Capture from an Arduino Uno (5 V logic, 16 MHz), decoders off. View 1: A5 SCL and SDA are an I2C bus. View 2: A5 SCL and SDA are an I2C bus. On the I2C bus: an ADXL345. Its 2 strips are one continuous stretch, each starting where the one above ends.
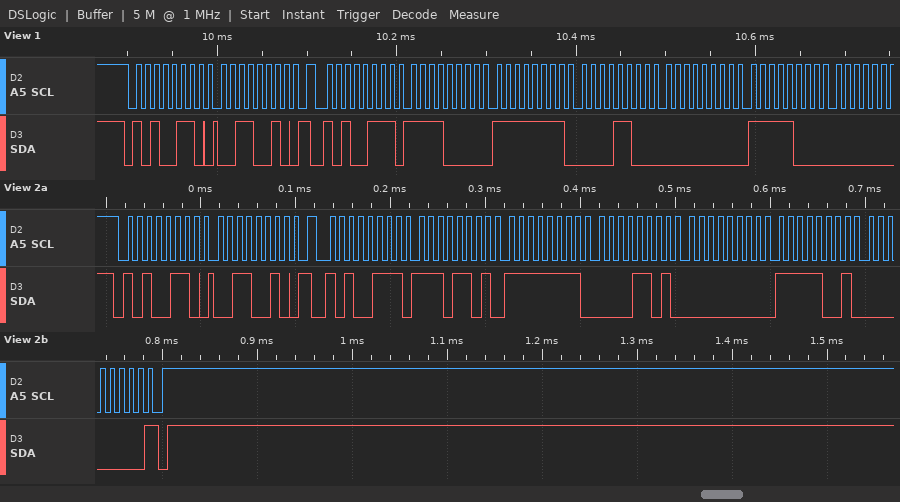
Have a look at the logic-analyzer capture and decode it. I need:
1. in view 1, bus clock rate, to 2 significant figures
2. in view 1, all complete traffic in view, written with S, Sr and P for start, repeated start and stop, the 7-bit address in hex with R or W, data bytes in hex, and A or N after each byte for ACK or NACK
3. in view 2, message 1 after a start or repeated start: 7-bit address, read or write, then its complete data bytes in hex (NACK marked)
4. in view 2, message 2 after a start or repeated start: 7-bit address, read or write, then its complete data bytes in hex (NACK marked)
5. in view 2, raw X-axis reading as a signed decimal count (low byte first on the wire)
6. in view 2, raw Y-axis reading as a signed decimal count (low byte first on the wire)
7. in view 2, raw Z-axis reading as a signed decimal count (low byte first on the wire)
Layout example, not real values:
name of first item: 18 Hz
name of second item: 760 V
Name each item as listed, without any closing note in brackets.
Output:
in view 1, bus clock rate, to 2 significant figures: 100 kHz
in view 1, all complete traffic in view, written with S, Sr and P for start, repeated start and stop, the 7-bit address in hex with R or W, data bytes in hex, and A or N after each byte for ACK or NACK: S 53W A 32 A Sr 53R A F0 A FF A 0C A 00 A F8 A
in view 2, message 1 after a start or repeated start: 7-bit address, read or write, then its complete data bytes in hex: 0x53 write: 32
in view 2, message 2 after a start or repeated start: 7-bit address, read or write, then its complete data bytes in hex: 0x53 read: ED FF 0D 00 F9 00 NACK
in view 2, raw X-axis reading as a signed decimal count: -19
in view 2, raw Y-axis reading as a signed decimal count: 13
in view 2, raw Z-axis reading as a signed decimal count: 249
